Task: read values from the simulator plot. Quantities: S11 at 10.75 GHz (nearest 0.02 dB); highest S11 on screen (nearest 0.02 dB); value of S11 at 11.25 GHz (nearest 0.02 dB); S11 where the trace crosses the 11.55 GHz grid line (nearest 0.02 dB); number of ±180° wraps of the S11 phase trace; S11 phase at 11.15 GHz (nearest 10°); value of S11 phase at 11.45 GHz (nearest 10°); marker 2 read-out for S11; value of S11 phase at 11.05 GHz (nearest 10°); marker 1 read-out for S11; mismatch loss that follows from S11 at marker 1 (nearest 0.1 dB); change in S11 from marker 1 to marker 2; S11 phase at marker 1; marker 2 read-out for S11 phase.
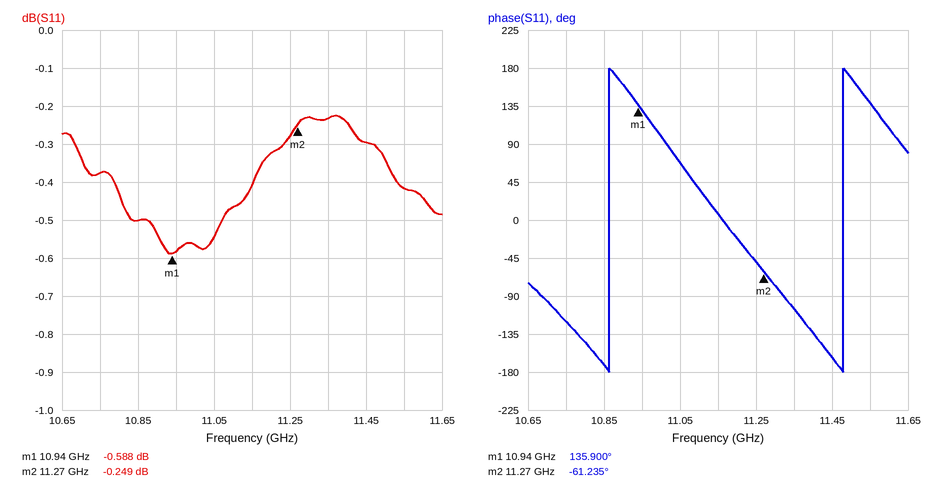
-0.38 dB
-0.22 dB
-0.28 dB
-0.42 dB
2
10°
-160°
-0.249 dB
70°
-0.588 dB
9.0 dB
0.339 dB
135.900°
-61.235°
